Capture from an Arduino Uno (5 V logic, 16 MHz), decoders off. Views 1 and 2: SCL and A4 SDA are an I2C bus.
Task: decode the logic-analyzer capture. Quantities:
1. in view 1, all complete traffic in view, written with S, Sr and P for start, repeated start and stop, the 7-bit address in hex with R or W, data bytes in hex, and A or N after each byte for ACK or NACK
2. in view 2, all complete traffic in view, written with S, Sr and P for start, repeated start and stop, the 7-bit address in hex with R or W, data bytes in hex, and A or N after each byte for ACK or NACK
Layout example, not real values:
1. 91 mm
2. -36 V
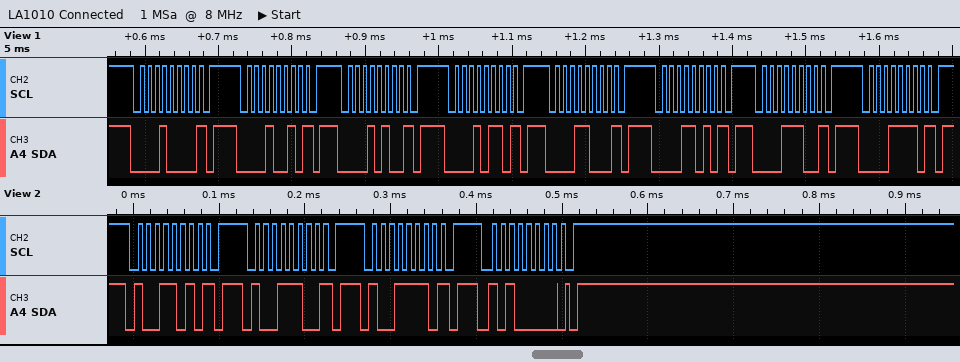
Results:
1. S 08W N P S 09W N P S 0AW N P S 0BW N P S 0CW N P S 0DW N P S 0EW N P S 0FW N P
2. S 4DW N P S 4EW N P S 4FW N P S 50W A P
